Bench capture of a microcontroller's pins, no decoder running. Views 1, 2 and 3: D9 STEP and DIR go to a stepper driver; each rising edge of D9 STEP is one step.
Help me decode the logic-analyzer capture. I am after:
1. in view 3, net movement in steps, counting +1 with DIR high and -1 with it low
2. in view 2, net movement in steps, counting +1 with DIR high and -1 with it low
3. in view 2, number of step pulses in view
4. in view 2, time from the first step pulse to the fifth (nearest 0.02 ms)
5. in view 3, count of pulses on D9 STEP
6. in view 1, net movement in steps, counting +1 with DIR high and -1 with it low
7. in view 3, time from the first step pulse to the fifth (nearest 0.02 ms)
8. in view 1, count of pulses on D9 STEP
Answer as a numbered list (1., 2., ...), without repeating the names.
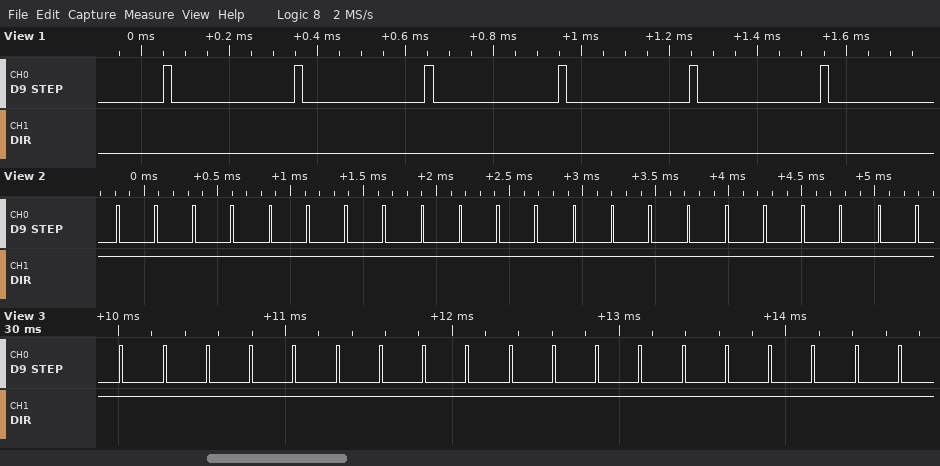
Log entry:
1. +19
2. +22
3. 22
4. 1.04 ms
5. 19
6. -6
7. 1.04 ms
8. 6
